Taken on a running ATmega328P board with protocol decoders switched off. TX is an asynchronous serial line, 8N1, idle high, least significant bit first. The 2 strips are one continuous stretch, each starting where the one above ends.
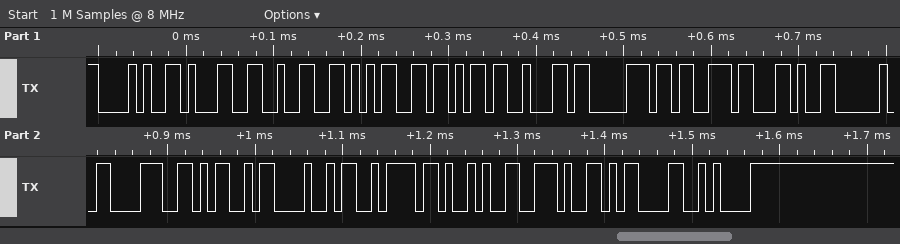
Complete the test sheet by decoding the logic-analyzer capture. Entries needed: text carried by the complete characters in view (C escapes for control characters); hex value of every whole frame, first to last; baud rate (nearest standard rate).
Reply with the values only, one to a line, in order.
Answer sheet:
"(125kbps, 8MHz).\r\n"
28 31 32 35 6B 62 70 73 2C 20 38 4D 48 7A 29 2E 0D 0A
115200 baud
